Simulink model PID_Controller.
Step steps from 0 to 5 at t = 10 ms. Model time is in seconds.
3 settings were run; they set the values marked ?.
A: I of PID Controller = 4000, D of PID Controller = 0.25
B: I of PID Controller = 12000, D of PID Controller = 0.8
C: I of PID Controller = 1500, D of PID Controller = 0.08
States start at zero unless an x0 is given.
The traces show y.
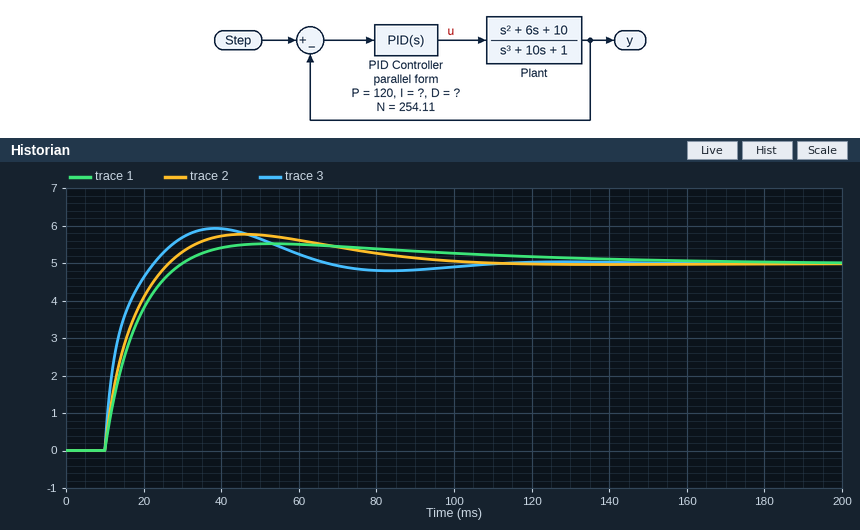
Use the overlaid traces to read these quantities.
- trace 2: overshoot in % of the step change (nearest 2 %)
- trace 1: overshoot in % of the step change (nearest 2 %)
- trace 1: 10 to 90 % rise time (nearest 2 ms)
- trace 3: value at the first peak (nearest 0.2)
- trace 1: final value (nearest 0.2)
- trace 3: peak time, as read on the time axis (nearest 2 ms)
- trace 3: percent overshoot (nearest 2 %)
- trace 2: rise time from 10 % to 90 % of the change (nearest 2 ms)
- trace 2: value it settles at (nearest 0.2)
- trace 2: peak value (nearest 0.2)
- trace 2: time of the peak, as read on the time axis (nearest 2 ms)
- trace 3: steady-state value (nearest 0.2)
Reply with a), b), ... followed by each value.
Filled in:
a) 16 %
b) 10 %
c) 14 ms
d) 6.0
e) 5.0
f) 38 ms
g) 18 %
h) 12 ms
i) 5.0
j) 5.8
k) 46 ms
l) 5.0
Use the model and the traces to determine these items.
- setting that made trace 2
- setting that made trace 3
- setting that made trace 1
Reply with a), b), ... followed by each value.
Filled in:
a) A
b) B
c) C
